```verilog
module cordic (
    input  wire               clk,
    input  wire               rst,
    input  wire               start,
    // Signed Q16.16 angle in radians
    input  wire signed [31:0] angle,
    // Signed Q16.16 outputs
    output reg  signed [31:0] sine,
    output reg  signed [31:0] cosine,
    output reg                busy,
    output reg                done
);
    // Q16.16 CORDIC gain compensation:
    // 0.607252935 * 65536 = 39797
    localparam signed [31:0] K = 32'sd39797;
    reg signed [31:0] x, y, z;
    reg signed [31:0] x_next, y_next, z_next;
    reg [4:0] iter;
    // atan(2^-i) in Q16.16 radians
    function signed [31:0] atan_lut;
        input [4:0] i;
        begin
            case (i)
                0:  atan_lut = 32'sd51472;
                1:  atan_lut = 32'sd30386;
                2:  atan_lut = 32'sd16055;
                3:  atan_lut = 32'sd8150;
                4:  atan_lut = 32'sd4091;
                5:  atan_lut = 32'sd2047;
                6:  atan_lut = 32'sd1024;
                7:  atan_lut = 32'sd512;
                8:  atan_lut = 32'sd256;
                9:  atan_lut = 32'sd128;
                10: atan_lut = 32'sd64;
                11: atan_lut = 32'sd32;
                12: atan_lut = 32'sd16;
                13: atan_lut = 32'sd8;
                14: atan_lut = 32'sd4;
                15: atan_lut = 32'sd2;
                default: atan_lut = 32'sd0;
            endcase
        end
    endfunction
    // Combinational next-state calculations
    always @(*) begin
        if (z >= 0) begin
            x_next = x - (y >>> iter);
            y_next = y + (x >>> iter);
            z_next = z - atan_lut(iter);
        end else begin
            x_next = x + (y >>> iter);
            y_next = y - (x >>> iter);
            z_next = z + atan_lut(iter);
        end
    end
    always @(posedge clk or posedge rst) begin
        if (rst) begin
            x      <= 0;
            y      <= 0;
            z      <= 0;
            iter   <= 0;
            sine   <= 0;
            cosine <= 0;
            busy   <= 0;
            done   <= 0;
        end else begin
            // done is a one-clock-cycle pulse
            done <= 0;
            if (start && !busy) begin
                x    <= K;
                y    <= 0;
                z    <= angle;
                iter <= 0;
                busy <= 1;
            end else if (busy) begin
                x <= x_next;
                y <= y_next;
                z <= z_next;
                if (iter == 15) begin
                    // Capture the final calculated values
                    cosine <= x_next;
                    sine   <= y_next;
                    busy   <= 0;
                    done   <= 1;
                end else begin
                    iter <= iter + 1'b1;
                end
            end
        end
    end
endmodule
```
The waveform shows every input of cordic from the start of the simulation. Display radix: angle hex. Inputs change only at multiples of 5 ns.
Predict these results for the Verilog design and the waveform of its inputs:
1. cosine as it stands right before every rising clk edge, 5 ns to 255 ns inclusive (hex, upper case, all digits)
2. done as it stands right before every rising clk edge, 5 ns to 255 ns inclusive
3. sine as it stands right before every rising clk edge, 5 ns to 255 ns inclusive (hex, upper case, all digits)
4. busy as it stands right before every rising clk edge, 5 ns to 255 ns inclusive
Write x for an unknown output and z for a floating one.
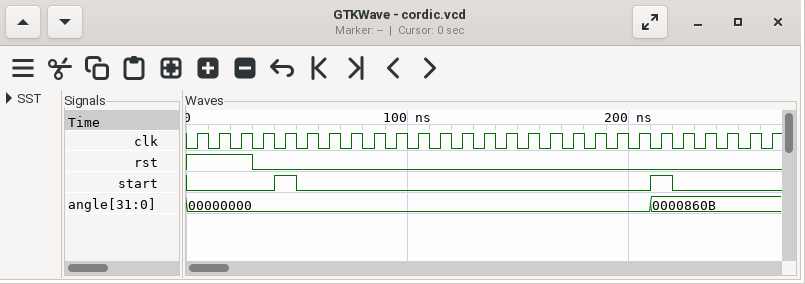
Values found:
00000000, 00000000, 00000000, 00000000, 00000000, 00000000, 00000000, 00000000, 00000000, 00000000, 00000000, 00000000, 00000000, 00000000, 00000000, 00000000, 00000000, 00000000, 00000000, 00000000, 00000000, 00010000, 00010000, 00010000, 00010000, 00010000
0 0 0 0 0 0 0 0 0 0 0 0 0 0 0 0 0 0 0 0 0 1 0 0 0 0
00000000, 00000000, 00000000, 00000000, 00000000, 00000000, 00000000, 00000000, 00000000, 00000000, 00000000, 00000000, 00000000, 00000000, 00000000, 00000000, 00000000, 00000000, 00000000, 00000000, 00000000, 00000002, 00000002, 00000002, 00000002, 00000002
0 0 0 0 0 1 1 1 1 1 1 1 1 1 1 1 1 1 1 1 1 0 1 1 1 1
